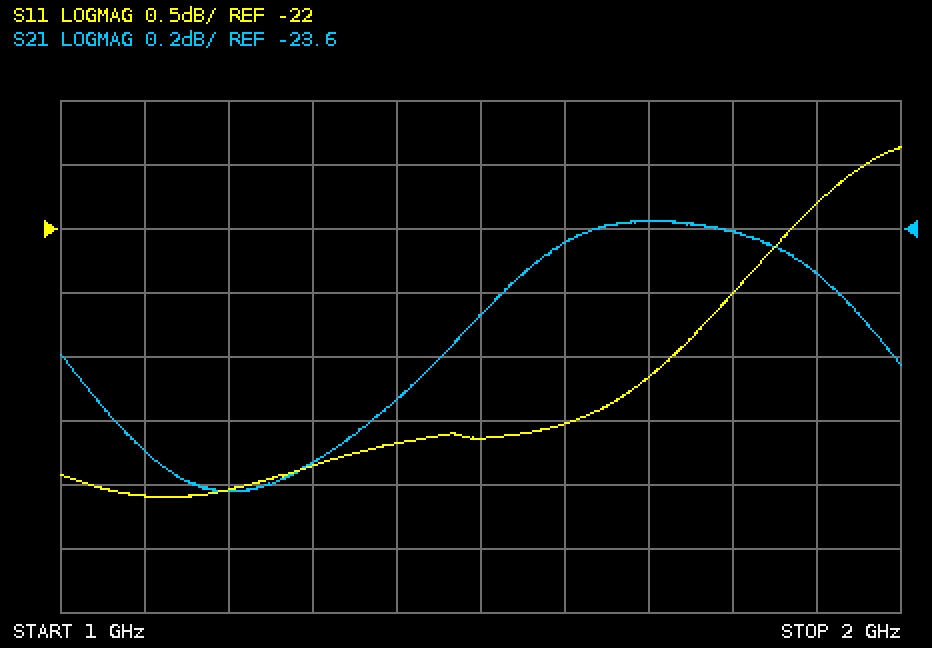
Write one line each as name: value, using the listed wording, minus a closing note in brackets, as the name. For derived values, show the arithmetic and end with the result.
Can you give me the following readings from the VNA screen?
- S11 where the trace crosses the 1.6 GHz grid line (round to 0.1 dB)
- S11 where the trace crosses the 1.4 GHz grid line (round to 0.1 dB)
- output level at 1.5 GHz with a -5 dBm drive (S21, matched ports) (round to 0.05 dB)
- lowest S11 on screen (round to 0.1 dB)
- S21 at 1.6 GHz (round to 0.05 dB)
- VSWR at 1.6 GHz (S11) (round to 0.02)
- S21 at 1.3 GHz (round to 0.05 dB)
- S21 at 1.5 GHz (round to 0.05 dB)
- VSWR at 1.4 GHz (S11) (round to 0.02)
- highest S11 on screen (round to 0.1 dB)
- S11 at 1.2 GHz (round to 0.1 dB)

S11 where the trace crosses the 1.6 GHz grid line: -23.5 dB
S11 where the trace crosses the 1.4 GHz grid line: -23.7 dB
output level at 1.5 GHz with a -5 dBm drive (S21, matched ports): -5 dBm + (-23.85 dB) = -28.85 dBm
lowest S11 on screen: -24.1 dB
S21 at 1.6 GHz: -23.65 dB
VSWR at 1.6 GHz (S11): |Γ| = 10^(-23.5/20) = 0.0668; VSWR = (1 + 0.0668)/(1 − 0.0668) ≈ 1.14
S21 at 1.3 GHz: -24.35 dB
S21 at 1.5 GHz: -23.85 dB
VSWR at 1.4 GHz (S11): |Γ| = 10^(-23.7/20) = 0.0653; VSWR = (1 + 0.0653)/(1 − 0.0653) ≈ 1.14
highest S11 on screen: -21.4 dB
S11 at 1.2 GHz: -24.0 dB
